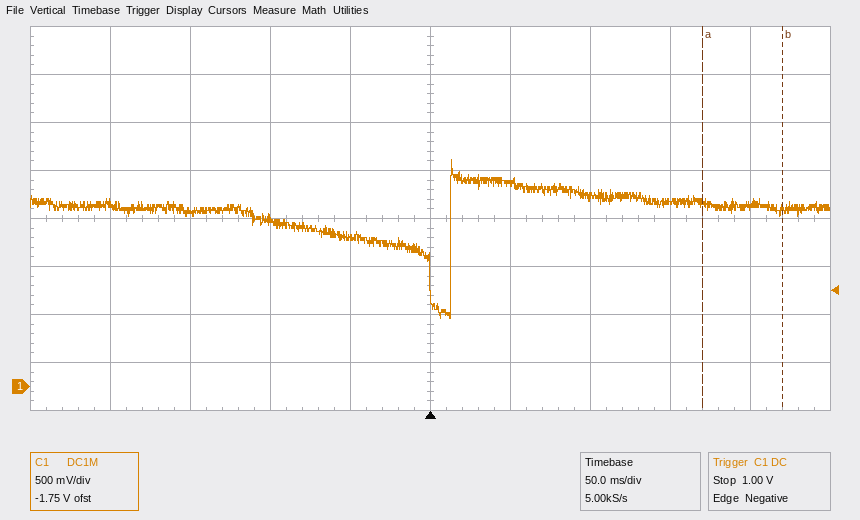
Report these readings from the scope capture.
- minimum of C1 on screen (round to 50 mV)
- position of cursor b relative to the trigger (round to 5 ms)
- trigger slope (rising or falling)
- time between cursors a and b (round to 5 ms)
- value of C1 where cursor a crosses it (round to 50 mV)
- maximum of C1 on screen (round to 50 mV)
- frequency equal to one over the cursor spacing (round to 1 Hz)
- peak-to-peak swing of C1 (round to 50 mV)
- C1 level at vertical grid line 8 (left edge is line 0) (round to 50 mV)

700 mV
+220 ms
falling
50 ms
1.90 V
2.35 V
20 Hz
1.65 V
1.95 V
